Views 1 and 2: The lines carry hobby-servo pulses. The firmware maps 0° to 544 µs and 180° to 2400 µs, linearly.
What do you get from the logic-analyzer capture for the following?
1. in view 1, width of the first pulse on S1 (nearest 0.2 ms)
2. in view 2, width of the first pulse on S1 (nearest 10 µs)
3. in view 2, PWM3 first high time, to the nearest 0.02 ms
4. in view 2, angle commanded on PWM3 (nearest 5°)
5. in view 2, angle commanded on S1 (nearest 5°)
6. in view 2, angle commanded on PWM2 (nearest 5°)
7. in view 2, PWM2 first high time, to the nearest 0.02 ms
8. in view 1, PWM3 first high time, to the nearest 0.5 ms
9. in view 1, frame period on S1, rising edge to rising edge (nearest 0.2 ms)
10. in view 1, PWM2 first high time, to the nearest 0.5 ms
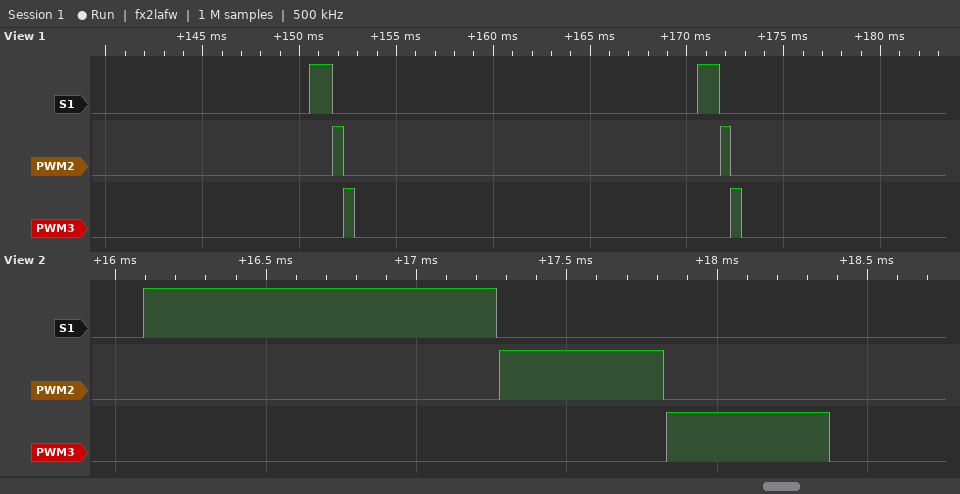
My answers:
1.2 ms
1170 µs
0.54 ms
0°
60°
0°
0.54 ms
0.5 ms
20.0 ms
0.5 ms
